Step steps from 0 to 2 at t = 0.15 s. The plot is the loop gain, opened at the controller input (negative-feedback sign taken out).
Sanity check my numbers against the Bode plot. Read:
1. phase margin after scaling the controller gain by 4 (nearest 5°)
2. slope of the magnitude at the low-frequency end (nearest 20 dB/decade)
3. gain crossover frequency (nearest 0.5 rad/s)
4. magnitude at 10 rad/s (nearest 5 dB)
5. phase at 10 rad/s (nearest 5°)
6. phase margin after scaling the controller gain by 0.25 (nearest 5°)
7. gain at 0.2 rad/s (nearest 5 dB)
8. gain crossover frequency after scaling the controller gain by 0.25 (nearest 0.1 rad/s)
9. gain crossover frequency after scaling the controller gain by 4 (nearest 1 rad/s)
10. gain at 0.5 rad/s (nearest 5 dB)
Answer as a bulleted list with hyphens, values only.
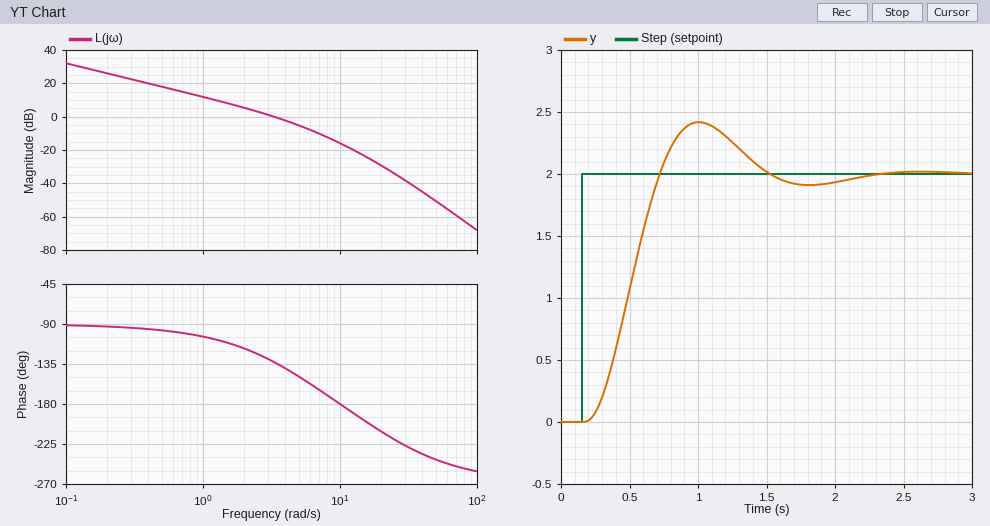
- 10°
- -20 dB/decade
- 3.5 rad/s
- -15 dB
- -180°
- 75°
- 25 dB
- 1.0 rad/s
- 8 rad/s
- 20 dB
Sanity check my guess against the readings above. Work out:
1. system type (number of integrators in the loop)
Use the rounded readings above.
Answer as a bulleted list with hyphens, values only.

- 1
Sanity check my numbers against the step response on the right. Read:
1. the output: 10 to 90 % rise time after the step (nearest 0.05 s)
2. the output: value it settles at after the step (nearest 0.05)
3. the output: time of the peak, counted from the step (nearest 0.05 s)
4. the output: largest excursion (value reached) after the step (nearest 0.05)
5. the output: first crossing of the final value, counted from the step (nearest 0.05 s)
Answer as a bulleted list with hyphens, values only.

- 0.35 s
- 2.00
- 0.85 s
- 2.40
- 0.55 s
